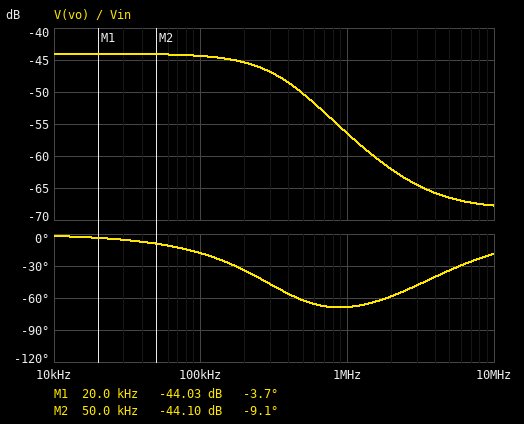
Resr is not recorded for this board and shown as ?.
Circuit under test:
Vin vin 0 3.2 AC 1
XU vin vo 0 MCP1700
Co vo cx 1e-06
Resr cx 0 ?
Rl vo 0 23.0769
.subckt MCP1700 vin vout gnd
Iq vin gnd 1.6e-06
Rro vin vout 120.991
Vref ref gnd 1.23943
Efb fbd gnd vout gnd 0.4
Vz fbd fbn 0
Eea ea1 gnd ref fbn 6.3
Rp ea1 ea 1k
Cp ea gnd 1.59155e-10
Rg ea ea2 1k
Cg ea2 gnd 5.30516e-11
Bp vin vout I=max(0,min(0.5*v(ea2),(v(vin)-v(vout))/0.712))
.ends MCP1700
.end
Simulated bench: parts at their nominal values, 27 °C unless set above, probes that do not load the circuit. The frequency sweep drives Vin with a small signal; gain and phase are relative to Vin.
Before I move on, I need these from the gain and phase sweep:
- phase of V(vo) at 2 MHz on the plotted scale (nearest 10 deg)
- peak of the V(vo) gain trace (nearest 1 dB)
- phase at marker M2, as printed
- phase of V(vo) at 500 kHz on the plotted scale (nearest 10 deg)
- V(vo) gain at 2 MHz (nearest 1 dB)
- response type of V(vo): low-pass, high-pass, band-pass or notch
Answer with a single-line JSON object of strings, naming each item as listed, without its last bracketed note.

{"phase of V(vo) at 2 MHz on the plotted scale": "-60 deg", "peak of the V(vo) gain trace": "-44 dB", "phase at marker M2, as printed": "-9.1 deg", "phase of V(vo) at 500 kHz on the plotted scale": "-60 deg", "V(vo) gain at 2 MHz": "-62 dB", "response type of V(vo): low-pass, high-pass, band-pass or notch": "low-pass"}
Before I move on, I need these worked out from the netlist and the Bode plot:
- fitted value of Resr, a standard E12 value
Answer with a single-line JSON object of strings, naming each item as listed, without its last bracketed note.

{"fitted value of Resr, a standard E12 value": "0.047 Ω"}
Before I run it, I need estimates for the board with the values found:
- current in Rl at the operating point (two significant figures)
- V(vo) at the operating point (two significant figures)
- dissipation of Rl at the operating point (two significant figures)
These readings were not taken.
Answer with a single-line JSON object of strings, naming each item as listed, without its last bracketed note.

{"current in Rl at the operating point": "130 mA", "V(vo) at the operating point": "3.0 V", "dissipation of Rl at the operating point": "390 mW"}
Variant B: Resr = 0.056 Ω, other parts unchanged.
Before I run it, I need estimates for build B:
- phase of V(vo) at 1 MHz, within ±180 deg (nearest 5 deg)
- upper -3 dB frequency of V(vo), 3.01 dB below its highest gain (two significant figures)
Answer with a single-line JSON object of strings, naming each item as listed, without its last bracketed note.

{"phase of V(vo) at 1 MHz, within ±180 deg": "-65 deg", "upper -3 dB frequency of V(vo), 3.01 dB below its highest gain": "300 kHz"}
